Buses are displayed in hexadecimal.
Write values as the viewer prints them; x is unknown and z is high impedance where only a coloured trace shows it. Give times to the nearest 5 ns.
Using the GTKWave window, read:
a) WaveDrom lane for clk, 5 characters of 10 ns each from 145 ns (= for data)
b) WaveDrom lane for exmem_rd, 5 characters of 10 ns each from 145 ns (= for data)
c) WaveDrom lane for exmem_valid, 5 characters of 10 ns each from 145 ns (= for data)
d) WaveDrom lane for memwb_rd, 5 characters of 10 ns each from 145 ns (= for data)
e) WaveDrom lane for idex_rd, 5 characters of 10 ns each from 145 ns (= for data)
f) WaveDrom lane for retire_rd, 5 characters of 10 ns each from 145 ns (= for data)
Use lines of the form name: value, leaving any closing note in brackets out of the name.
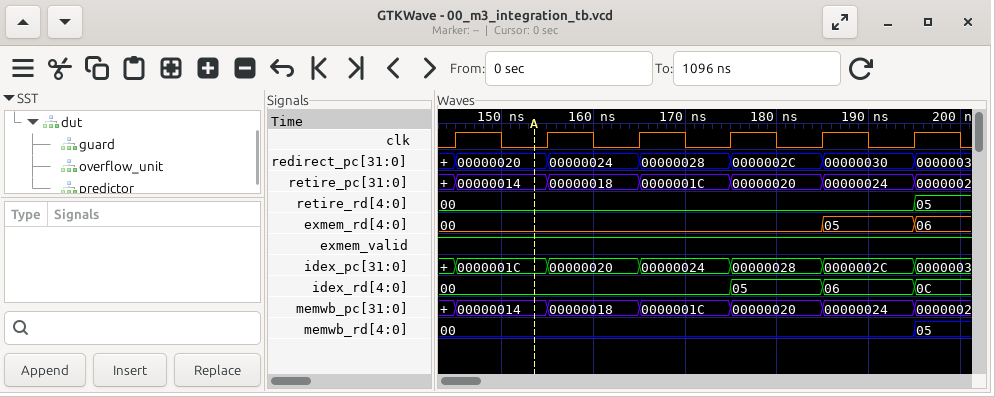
WaveDrom lane for clk, 5 characters of 10 ns each from 145 ns: {name: 'clk', wave: 'p....'}
WaveDrom lane for exmem_rd, 5 characters of 10 ns each from 145 ns: {name: 'exmem_rd', wave: '=...=', data: '00 05'}
WaveDrom lane for exmem_valid, 5 characters of 10 ns each from 145 ns: {name: 'exmem_valid', wave: '1....'}
WaveDrom lane for memwb_rd, 5 characters of 10 ns each from 145 ns: {name: 'memwb_rd', wave: '=....', data: '00'}
WaveDrom lane for idex_rd, 5 characters of 10 ns each from 145 ns: {name: 'idex_rd', wave: '=..==', data: '00 05 06'}
WaveDrom lane for retire_rd, 5 characters of 10 ns each from 145 ns: {name: 'retire_rd', wave: '=....', data: '00'}
